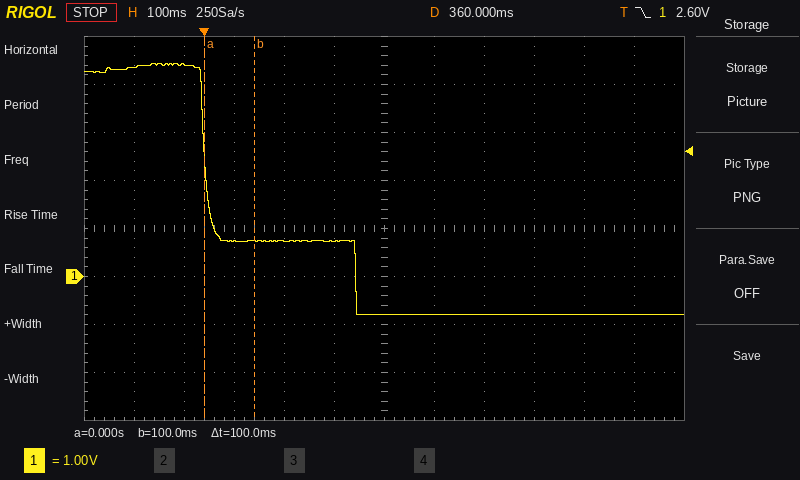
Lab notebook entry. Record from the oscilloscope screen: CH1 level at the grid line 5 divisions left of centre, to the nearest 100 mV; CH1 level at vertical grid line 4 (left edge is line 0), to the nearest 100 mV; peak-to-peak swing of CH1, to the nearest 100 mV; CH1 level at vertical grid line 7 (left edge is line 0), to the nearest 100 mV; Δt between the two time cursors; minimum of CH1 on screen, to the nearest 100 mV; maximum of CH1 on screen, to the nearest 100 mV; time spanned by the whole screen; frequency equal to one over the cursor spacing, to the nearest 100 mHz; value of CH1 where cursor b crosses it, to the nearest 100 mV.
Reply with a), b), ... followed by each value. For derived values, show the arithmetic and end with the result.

a) 4.4 V
b) 700 mV
c) 4.4 V − (-800 mV) = 5.2 V
d) -800 mV
e) 100 ms
f) -800 mV
g) 4.4 V
h) 1.2 s
i) 1 / 100 ms ≈ 10.0 Hz
j) 700 mV
